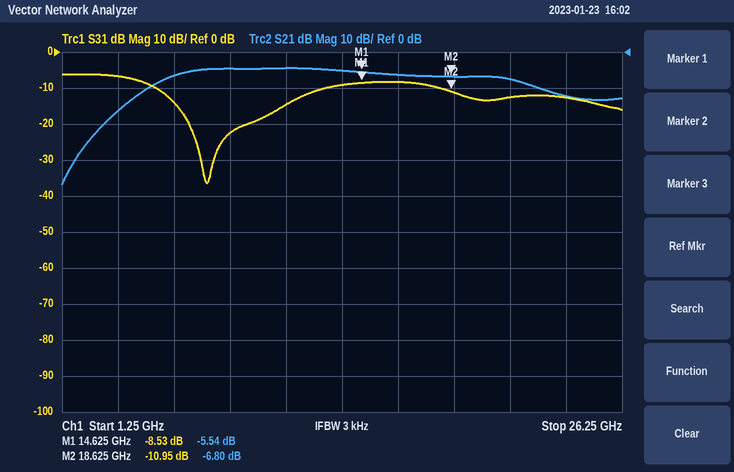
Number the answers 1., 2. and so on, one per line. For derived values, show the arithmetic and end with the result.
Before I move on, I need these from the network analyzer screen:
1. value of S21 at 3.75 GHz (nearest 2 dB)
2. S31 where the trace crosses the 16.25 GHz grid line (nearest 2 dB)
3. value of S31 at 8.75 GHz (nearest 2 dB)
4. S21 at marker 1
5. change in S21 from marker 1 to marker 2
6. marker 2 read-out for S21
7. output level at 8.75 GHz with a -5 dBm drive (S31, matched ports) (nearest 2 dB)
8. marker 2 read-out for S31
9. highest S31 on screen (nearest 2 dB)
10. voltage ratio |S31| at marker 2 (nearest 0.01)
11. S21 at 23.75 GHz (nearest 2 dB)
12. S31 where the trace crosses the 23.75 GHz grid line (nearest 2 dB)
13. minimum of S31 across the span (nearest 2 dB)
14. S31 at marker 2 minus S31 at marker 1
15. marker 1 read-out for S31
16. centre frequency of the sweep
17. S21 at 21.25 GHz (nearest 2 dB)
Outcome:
1. -16 dB
2. -8 dB
3. -22 dB
4. -5.54 dB
5. -6.8 − (-5.54) = -1.26 dB
6. -6.80 dB
7. -5 dBm + (-22 dB) = -28 dBm
8. -10.95 dB
9. -6 dB
10. 10^(-10.95/20) ≈ 0.28
11. -12 dB
12. -12 dB
13. -36 dB
14. -10.95 − (-8.53) = -2.42 dB
15. -8.53 dB
16. 13.75 GHz
17. -8 dB
